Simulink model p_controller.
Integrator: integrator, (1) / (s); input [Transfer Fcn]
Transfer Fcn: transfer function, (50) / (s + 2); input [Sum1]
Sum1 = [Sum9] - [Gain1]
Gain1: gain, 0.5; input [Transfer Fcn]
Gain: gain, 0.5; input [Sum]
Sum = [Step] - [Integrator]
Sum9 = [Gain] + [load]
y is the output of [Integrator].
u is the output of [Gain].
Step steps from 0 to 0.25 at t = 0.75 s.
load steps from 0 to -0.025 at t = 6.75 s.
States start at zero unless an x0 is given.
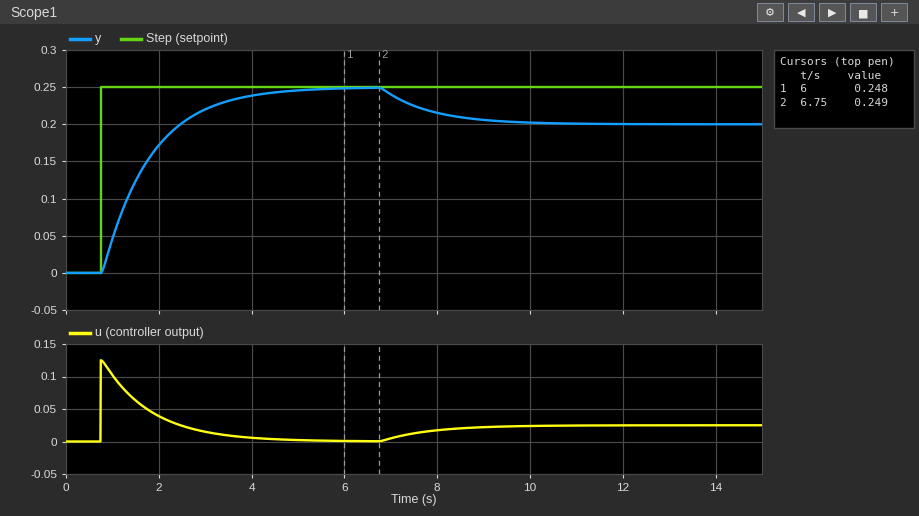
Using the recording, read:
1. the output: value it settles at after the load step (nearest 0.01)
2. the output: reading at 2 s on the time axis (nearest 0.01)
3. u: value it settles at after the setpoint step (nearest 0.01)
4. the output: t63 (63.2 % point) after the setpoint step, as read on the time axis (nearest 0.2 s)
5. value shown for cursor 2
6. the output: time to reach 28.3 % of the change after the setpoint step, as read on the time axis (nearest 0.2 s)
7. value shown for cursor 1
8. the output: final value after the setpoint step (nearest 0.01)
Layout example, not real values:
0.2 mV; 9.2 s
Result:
0.20; 0.17; 0.00; 1.8 s; 0.249; 1.2 s; 0.248; 0.25
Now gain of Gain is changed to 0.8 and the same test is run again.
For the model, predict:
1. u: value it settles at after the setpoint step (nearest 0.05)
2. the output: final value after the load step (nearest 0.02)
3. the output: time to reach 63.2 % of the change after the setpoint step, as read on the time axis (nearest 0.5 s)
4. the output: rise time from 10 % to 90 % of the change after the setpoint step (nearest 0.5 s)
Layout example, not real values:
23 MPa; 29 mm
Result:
0.00; 0.22; 1.5 s; 1.5 s
